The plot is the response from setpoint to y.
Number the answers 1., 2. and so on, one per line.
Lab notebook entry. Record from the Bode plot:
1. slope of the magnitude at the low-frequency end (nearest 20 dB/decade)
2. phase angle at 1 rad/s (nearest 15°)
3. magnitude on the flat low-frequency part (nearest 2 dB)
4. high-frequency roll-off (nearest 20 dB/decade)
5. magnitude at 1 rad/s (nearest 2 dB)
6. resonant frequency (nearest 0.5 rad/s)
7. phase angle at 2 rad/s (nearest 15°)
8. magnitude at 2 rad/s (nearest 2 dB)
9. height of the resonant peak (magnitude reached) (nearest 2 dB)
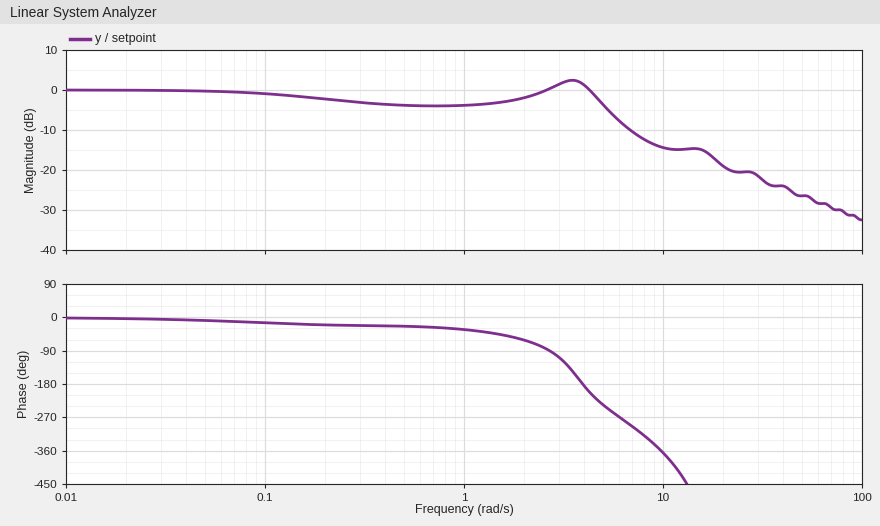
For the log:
1. 0 dB/decade
2. -30°
3. 0 dB
4. -20 dB/decade
5. -4 dB
6. 3.5 rad/s
7. -60°
8. -2 dB
9. 2 dB
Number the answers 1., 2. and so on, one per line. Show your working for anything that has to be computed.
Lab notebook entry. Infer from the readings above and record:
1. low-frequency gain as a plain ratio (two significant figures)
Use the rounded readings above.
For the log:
1. 10^(0 / 20) = 1.0
